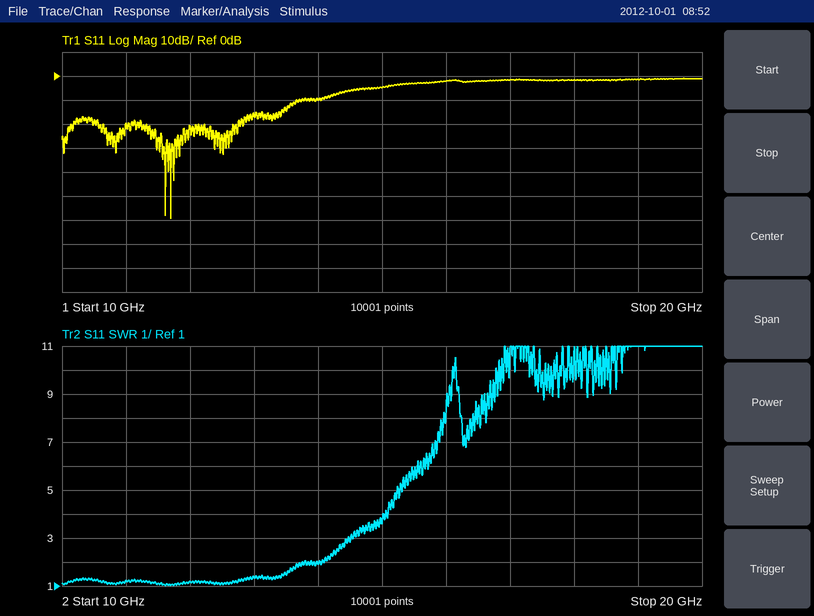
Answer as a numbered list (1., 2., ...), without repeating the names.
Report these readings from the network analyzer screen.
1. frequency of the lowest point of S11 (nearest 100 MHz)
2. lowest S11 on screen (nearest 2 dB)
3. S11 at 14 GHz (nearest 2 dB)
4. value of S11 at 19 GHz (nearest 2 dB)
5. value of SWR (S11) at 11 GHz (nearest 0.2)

1. 11.7 GHz
2. -60 dB
3. -10 dB
4. -2 dB
5. 1.2
